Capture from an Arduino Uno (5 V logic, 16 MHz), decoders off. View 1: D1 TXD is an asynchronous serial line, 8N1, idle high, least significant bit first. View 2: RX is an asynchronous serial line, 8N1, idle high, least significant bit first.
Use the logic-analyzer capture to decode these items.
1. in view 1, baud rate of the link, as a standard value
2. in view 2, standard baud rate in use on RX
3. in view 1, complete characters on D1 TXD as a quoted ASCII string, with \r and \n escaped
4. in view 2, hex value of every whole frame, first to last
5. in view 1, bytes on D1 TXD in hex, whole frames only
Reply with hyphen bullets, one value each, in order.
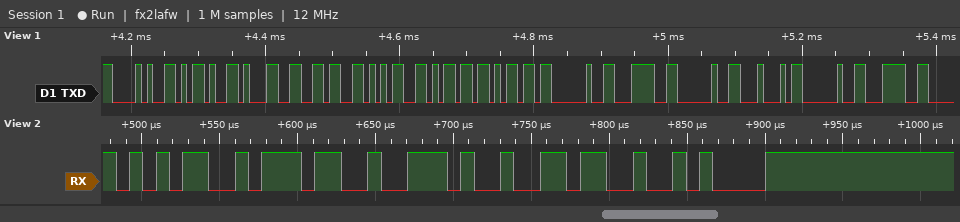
- 115200 baud
- 115200 baud
- "(-165mm < D <"
- 35 37 2E 36 0A
- 28 2D 31 36 35 6D 6D 20 3C 20 44 20 3C
